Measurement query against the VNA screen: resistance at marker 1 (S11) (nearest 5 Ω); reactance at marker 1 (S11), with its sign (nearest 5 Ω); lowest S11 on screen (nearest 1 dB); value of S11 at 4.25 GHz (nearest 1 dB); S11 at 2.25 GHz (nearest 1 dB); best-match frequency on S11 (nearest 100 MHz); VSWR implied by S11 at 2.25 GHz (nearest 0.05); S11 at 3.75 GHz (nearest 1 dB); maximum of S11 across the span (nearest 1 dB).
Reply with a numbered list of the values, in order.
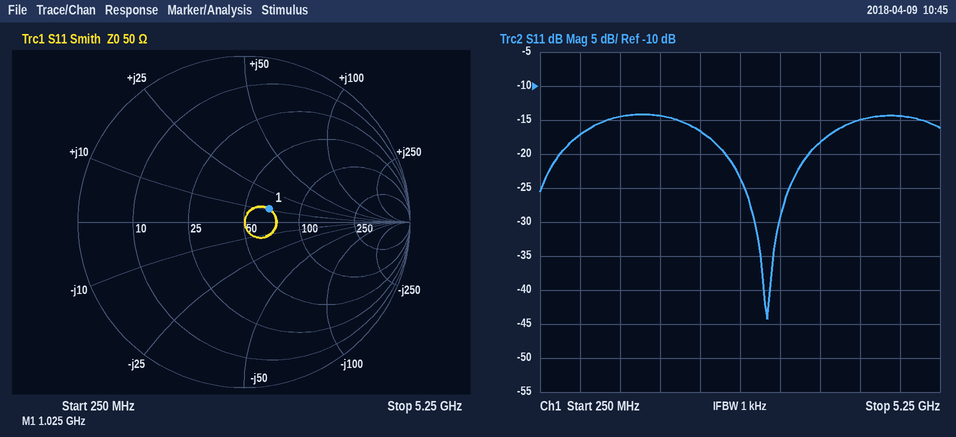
1. 65 Ω
2. +10 Ω
3. -44 dB
4. -15 dB
5. -17 dB
6. 3.1 GHz
7. 1.35
8. -18 dB
9. -14 dB
